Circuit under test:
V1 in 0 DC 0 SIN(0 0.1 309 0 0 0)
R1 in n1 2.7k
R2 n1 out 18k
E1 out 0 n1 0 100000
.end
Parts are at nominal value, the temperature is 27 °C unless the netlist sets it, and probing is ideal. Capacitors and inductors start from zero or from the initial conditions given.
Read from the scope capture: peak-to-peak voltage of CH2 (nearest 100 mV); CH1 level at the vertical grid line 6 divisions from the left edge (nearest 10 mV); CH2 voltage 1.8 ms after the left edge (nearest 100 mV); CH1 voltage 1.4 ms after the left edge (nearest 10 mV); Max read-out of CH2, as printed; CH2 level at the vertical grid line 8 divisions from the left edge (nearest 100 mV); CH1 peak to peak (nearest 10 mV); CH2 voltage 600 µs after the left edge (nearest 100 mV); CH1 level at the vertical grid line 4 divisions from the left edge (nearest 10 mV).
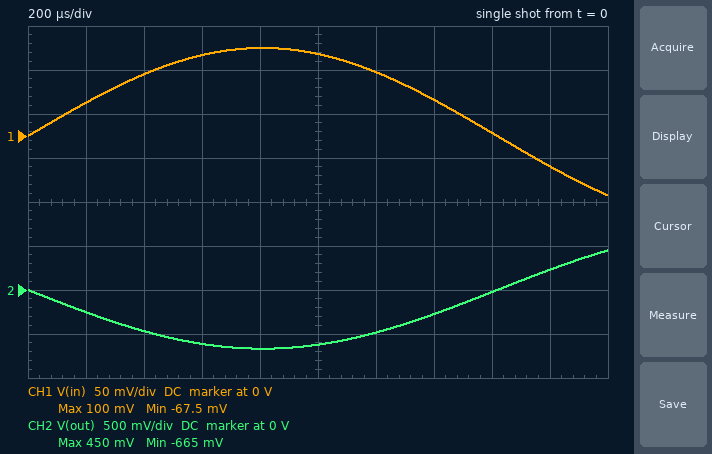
1.1 V
70 mV
200 mV
40 mV
450 mV
0 V
170 mV
-600 mV
100 mV
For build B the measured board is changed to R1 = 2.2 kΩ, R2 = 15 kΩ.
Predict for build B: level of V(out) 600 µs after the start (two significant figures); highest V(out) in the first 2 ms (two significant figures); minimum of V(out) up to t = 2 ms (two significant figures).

-630 mV
460 mV
-680 mV
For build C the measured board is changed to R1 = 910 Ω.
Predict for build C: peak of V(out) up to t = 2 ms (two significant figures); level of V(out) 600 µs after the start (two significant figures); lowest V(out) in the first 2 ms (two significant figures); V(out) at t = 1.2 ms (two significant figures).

1.3 V
-1.8 V
-2.0 V
-1.4 V
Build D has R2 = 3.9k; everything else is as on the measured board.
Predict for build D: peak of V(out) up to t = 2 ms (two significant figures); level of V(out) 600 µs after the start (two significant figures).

98 mV
-130 mV
